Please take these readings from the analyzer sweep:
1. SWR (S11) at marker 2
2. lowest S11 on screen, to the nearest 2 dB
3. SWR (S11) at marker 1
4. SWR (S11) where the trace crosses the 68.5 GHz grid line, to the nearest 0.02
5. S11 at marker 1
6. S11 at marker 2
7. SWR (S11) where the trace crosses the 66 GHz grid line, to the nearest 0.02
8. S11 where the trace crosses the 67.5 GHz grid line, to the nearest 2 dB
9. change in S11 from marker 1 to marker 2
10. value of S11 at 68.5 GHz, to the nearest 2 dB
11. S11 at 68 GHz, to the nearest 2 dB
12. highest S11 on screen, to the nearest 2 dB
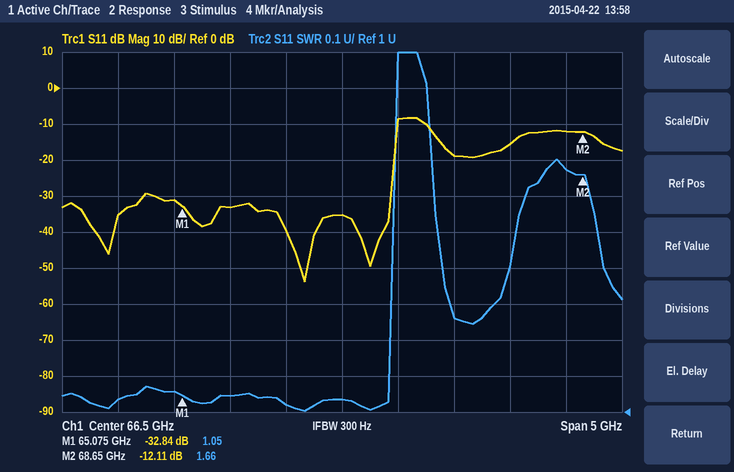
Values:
1.66
-54 dB
1.05
1.68
-32.84 dB
-12.11 dB
1.02
-18 dB
20.73 dB
-12 dB
-16 dB
-8 dB
